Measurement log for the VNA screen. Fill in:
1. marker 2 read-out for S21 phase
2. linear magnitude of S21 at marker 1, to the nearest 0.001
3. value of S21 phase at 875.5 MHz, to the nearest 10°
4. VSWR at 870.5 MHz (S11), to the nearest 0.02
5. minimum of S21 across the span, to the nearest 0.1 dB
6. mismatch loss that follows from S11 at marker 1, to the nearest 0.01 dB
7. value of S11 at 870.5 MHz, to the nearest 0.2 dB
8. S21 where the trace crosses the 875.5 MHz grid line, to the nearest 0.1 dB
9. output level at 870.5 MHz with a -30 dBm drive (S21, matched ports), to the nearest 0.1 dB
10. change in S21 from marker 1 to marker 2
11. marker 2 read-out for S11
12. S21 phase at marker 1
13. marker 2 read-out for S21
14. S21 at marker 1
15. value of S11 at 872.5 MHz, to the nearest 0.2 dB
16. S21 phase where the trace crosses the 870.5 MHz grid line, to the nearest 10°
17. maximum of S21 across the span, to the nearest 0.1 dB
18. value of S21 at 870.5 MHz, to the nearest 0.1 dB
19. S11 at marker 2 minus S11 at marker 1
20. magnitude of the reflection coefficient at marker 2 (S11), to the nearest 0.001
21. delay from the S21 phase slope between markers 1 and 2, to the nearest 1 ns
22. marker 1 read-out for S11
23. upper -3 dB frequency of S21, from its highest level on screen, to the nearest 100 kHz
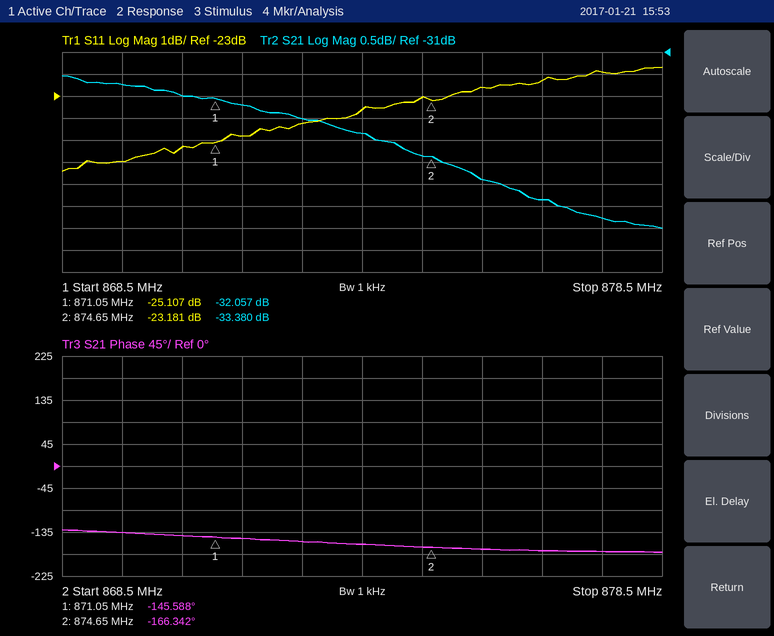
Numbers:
-166.342°
0.025
-170°
1.12
-35.0 dB
0.01 dB
-25.4 dB
-33.9 dB
-62.0 dBm
-1.323 dB
-23.181 dB
-145.588°
-33.380 dB
-32.057 dB
-24.2 dB
-140°
-31.5 dB
-32.0 dB
1.926 dB
0.069
16 ns
-25.107 dB
876.9 MHz
